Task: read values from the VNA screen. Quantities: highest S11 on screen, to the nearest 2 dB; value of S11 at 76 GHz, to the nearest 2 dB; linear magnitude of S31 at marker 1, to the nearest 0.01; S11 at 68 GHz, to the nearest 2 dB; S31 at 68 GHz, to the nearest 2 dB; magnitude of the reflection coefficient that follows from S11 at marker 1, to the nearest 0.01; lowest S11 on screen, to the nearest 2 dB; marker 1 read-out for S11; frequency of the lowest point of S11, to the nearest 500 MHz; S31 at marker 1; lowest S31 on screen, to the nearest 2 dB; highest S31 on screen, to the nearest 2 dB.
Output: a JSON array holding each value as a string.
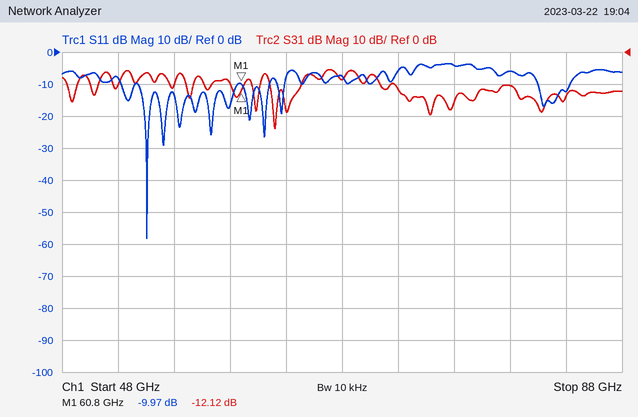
["-4 dB", "-4 dB", "0.25", "-8 dB", "-8 dB", "0.32", "-58 dB", "-9.97 dB", "54.0 GHz", "-12.12 dB", "-24 dB", "-6 dB"]
